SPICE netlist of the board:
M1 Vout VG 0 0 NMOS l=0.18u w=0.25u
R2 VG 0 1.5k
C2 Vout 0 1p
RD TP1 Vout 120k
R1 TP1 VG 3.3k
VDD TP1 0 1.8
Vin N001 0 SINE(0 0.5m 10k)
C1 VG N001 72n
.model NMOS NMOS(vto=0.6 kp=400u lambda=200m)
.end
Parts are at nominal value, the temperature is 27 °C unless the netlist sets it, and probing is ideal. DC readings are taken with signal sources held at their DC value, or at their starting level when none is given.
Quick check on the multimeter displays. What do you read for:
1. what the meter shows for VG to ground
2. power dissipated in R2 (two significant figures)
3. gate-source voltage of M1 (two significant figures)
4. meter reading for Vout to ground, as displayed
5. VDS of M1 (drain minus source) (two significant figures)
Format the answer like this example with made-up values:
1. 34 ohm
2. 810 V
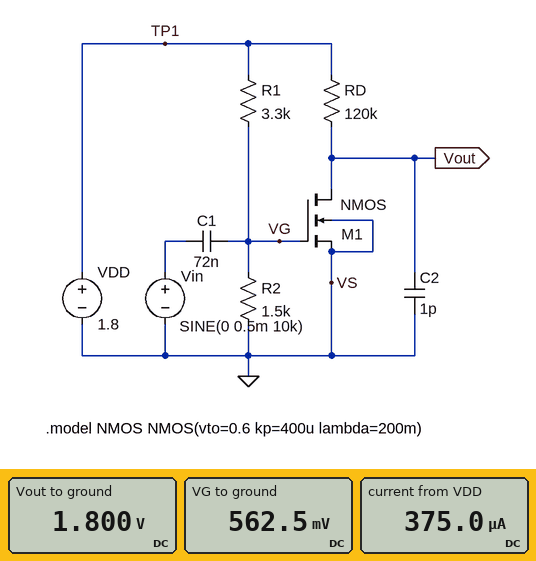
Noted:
1. 562.5 mV
2. 210 µW
3. 560 mV
4. 1.800 V
5. 1.8 V
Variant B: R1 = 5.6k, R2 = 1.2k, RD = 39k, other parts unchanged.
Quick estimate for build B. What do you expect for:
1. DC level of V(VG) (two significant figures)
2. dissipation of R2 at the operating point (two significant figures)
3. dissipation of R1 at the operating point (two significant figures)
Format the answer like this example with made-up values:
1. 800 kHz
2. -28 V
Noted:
1. 320 mV
2. 84 µW
3. 390 µW
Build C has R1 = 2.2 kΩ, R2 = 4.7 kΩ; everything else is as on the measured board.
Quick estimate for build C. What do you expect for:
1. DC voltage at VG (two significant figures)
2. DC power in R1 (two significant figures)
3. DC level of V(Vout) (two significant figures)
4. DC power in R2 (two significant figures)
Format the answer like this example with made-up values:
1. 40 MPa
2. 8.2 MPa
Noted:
1. 1.2 V
2. 150 µW
3. 43 mV
4. 320 µW
